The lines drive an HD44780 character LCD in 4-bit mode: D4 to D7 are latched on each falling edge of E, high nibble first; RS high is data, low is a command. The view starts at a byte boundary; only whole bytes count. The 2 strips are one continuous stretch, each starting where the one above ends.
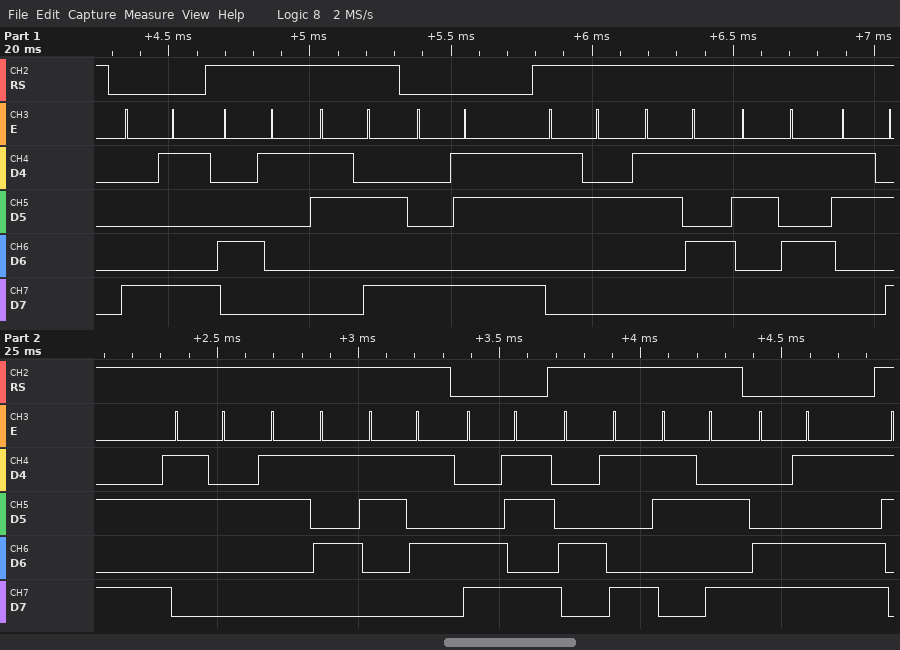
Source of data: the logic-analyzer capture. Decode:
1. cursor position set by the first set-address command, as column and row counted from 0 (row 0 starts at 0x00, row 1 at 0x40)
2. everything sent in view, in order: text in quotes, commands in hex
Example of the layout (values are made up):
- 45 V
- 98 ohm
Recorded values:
- column 9, row 0
- 0x89 "A:" 0x8B "255:255" 0xCB "I:" 0xCD
